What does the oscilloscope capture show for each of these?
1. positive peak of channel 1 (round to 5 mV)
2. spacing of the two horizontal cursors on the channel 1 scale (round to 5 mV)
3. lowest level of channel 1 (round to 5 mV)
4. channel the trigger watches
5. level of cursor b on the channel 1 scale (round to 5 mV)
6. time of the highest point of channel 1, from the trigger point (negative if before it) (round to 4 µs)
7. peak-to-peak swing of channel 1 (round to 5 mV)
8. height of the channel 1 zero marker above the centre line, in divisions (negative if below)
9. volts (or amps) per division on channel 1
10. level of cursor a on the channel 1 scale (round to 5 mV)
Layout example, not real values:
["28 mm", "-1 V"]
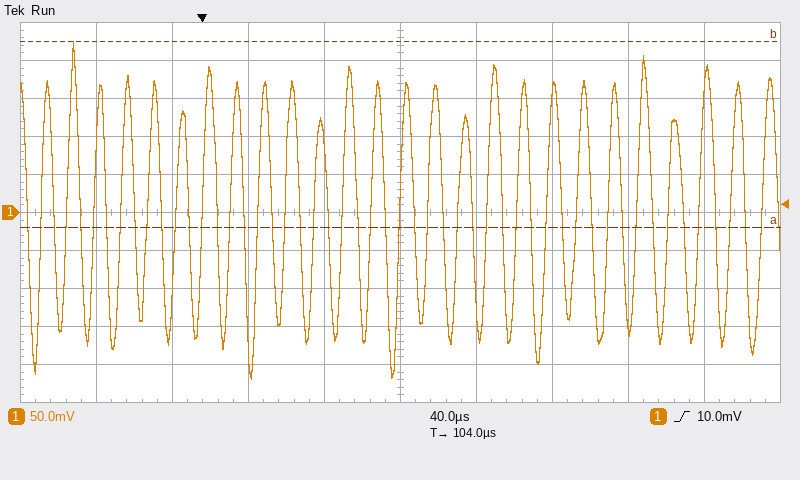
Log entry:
["225 mV", "245 mV", "-220 mV", "channel 1", "225 mV", "-68 µs", "445 mV", "0.0 div", "50 mV", "-20 mV"]
